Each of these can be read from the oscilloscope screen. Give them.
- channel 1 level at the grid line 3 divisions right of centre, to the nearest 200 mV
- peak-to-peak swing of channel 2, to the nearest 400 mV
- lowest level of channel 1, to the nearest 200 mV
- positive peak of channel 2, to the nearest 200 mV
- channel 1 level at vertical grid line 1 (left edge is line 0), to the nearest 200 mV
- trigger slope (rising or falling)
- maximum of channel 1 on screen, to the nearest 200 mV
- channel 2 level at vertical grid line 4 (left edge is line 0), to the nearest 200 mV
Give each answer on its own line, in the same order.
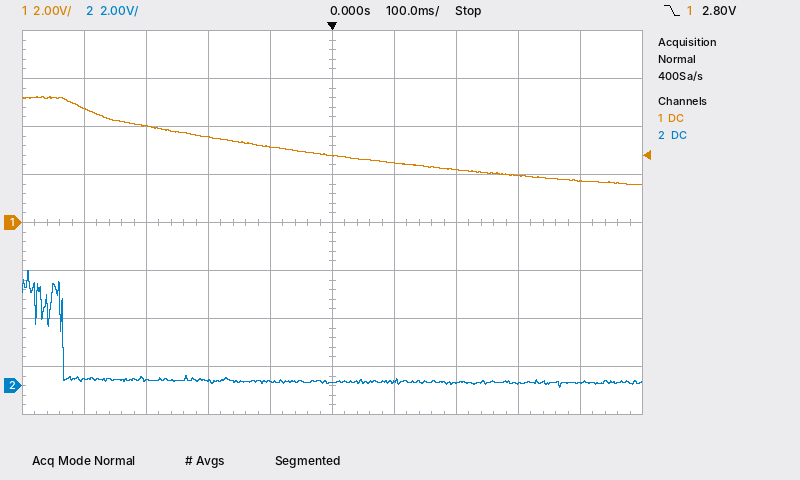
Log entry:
2.0 V
4.8 V
1.6 V
4.8 V
4.8 V
falling
5.2 V
200 mV
